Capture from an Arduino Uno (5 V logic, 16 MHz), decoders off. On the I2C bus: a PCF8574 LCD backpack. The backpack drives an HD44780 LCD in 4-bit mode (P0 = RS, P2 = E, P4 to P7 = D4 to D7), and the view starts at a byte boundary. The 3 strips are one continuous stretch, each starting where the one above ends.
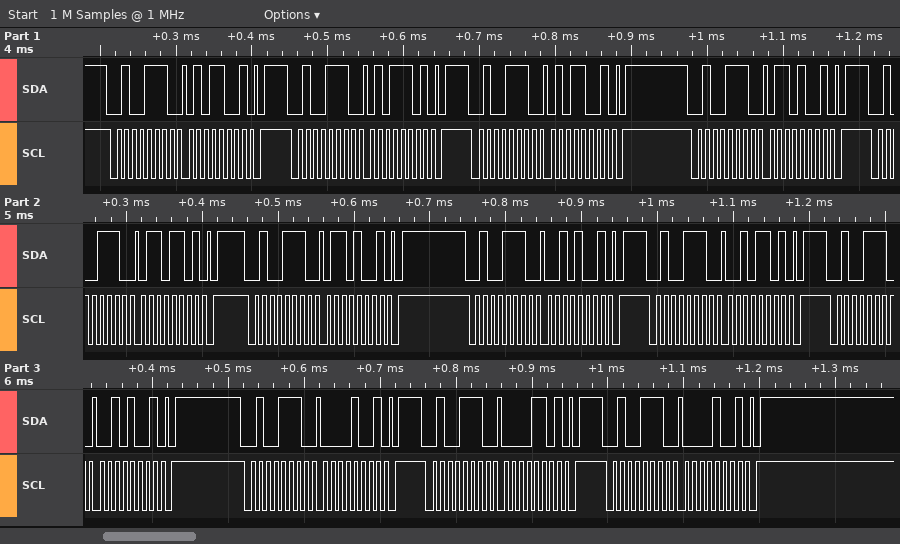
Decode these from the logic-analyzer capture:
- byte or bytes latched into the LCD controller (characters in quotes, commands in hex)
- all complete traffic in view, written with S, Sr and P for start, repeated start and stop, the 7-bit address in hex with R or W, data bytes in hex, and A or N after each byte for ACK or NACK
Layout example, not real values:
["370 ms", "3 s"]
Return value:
["'V' ' '", "S 27W A 59 A P S 27W A 5D A P S 27W A 59 A P S 27W A 69 A P S 27W A 6D A P S 27W A 69 A P S 27W A 29 A P S 27W A 2D A P S 27W A 29 A P S 27W A 09 A P S 27W A 0D A P S 27W A 09 A P"]
